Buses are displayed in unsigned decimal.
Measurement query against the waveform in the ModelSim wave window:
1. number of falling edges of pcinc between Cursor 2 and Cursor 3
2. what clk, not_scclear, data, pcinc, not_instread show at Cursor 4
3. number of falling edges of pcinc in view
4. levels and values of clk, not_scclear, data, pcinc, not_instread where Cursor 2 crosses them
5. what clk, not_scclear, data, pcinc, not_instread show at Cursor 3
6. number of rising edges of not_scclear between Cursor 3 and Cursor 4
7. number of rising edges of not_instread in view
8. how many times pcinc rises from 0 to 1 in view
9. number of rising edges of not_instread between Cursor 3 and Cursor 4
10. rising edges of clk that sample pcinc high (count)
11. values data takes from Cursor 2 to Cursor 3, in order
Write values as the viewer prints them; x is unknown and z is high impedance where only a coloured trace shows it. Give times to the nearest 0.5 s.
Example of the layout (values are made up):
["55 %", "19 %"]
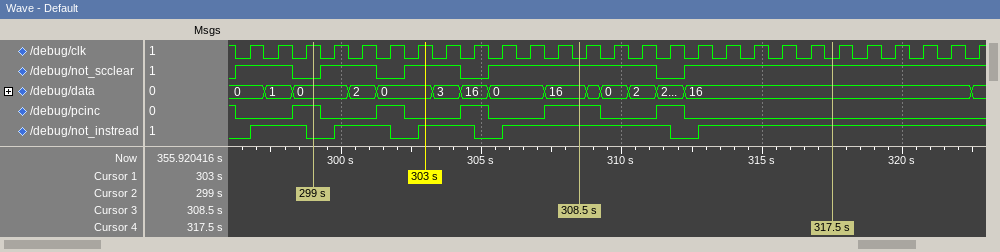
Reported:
["3", "clk=0, not_scclear=1, data=16, pcinc=0, not_instread=1", "6", "clk=1, not_scclear=0, data=0, pcinc=1, not_instread=0", "clk=0, not_scclear=1, data=16, pcinc=1, not_instread=1", "1", "5", "5", "1", "6", "0, 2, 0, 3, 16, 0, 16"]
